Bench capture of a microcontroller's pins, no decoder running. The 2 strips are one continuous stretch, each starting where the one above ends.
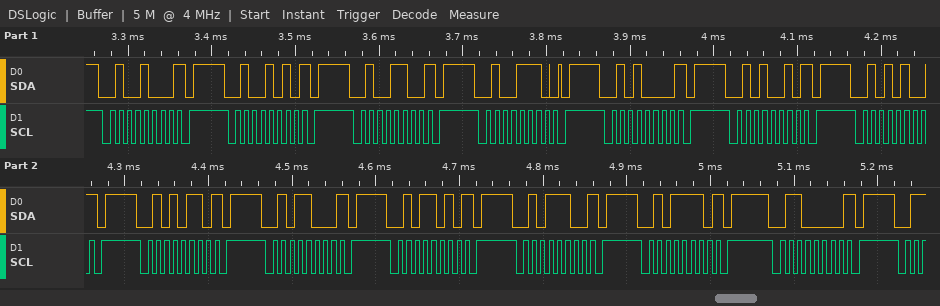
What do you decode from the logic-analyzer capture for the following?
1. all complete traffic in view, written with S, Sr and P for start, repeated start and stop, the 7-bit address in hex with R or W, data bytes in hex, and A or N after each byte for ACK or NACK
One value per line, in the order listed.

S 24W N P S 25W N P S 26W N P S 27W A P S 28W N P S 29W N P S 2AW N P S 2BW N P S 2CW N P S 2DW N P S 2EW N P S 2FW N P S 30W N P
